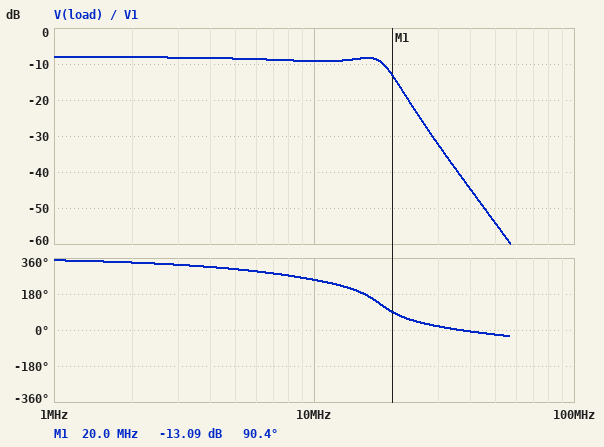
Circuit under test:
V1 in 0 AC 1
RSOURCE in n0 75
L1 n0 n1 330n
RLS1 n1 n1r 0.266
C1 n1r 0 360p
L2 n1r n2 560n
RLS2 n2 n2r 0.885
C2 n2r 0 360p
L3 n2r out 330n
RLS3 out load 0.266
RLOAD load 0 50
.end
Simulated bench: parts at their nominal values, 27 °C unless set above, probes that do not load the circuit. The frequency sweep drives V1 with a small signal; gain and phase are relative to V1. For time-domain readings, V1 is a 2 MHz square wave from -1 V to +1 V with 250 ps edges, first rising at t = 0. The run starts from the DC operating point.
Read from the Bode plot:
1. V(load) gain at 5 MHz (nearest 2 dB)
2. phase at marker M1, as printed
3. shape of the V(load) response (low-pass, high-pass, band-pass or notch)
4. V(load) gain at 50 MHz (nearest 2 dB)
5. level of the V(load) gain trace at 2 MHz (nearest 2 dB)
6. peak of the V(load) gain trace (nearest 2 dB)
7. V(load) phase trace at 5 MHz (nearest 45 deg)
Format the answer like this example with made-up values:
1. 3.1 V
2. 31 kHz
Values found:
1. -8 dB
2. 90.4 deg
3. low-pass
4. -54 dB
5. -8 dB
6. -8 dB
7. 315 deg
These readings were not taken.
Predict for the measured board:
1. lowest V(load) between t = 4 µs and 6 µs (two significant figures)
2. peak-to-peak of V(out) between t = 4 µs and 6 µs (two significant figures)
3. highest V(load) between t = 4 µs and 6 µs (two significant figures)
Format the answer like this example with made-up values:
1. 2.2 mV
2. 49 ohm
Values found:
1. -460 mV
2. 930 mV
3. 460 mV
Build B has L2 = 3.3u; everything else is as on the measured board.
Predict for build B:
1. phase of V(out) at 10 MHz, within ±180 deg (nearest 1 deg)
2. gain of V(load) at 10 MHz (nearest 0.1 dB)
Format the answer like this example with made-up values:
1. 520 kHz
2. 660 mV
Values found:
1. 154 deg
2. -16.7 dB
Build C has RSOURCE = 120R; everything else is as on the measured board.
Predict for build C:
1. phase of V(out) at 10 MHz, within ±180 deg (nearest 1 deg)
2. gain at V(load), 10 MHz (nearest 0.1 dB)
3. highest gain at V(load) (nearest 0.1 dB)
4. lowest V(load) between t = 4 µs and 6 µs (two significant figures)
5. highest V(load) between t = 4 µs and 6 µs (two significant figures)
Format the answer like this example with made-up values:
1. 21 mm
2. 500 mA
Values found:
1. -108 deg
2. -12.4 dB
3. -10.7 dB
4. -320 mV
5. 320 mV
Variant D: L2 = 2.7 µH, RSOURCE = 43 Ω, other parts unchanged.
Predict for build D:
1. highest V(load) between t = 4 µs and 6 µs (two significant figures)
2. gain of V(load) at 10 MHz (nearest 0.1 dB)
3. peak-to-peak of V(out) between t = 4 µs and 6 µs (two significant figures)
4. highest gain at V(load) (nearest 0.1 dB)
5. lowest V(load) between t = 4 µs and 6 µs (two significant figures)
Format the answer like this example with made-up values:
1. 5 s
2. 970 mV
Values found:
1. 530 mV
2. -11.4 dB
3. 1.1 V
4. -5.5 dB
5. -530 mV
